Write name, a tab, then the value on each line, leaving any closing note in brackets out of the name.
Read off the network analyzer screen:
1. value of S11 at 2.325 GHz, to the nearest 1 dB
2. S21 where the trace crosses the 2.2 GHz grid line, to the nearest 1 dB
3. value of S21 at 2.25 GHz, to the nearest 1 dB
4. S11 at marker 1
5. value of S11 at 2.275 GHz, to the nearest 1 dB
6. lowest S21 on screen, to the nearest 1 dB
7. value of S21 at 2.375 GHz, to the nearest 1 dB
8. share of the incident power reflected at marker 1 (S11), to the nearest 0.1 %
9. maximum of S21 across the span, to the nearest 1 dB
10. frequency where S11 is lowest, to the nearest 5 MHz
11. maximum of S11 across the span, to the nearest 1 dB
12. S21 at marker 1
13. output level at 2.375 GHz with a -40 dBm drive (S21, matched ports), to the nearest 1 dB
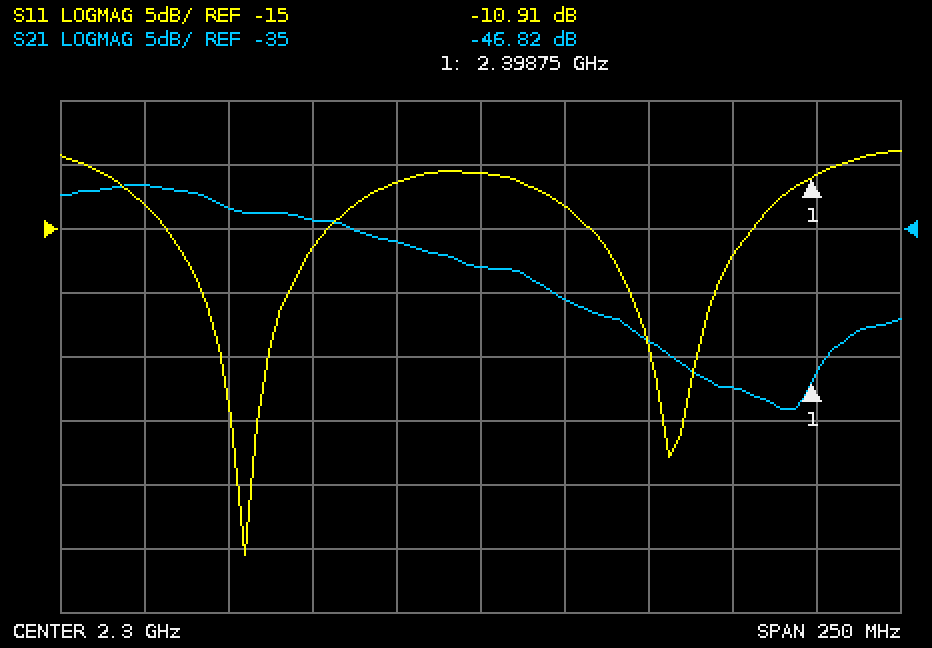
value of S11 at 2.325 GHz, to the nearest 1 dB	-13 dB
S21 where the trace crosses the 2.2 GHz grid line, to the nearest 1 dB	-32 dB
value of S21 at 2.25 GHz, to the nearest 1 dB	-34 dB
S11 at marker 1	-10.91 dB
value of S11 at 2.275 GHz, to the nearest 1 dB	-11 dB
lowest S21 on screen, to the nearest 1 dB	-49 dB
value of S21 at 2.375 GHz, to the nearest 1 dB	-47 dB
share of the incident power reflected at marker 1 (S11), to the nearest 0.1 %	8.1 %
maximum of S21 across the span, to the nearest 1 dB	-32 dB
frequency where S11 is lowest, to the nearest 5 MHz	2.230 GHz
maximum of S11 across the span, to the nearest 1 dB	-9 dB
S21 at marker 1	-46.82 dB
output level at 2.375 GHz with a -40 dBm drive (S21, matched ports), to the nearest 1 dB	-87 dBm
